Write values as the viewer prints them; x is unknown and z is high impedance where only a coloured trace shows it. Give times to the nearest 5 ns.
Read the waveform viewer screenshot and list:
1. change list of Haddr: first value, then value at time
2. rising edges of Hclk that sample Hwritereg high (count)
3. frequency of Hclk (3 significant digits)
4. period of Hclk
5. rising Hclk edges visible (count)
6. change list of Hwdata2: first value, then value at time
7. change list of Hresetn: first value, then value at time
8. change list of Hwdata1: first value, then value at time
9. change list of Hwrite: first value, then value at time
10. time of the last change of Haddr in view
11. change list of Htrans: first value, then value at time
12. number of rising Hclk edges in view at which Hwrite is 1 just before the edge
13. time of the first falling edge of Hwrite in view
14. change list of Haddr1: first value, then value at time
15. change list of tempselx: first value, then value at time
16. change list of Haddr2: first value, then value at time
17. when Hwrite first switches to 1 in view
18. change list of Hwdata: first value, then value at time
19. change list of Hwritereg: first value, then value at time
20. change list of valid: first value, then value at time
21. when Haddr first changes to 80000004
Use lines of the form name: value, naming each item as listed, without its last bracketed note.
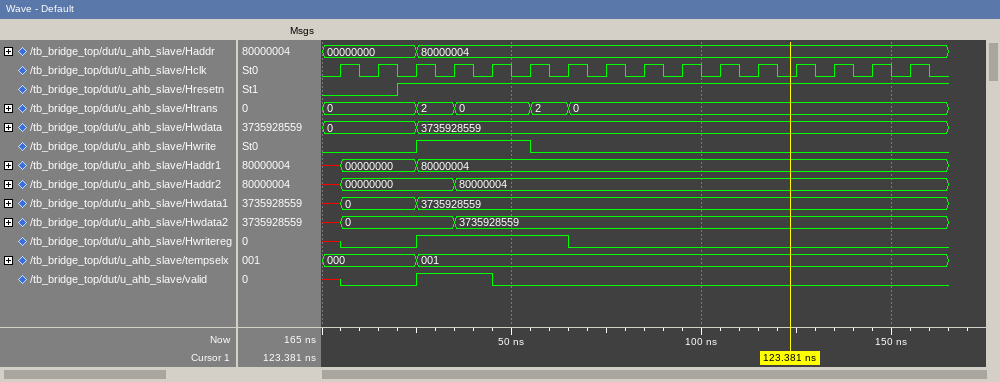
change list of Haddr: first value, then value at time: 00000000, 80000004 at 25 ns
rising edges of Hclk that sample Hwritereg high: 4
frequency of Hclk: 100 MHz
period of Hclk: 10 ns
rising Hclk edges visible: 16
change list of Hwdata2: first value, then value at time: x, 0 at 5 ns, 3735928559 at 35 ns
change list of Hresetn: first value, then value at time: 0, 1 at 20 ns
change list of Hwdata1: first value, then value at time: x, 0 at 5 ns, 3735928559 at 25 ns
change list of Hwrite: first value, then value at time: 0, 1 at 25 ns, 0 at 55 ns
time of the last change of Haddr in view: 25 ns
change list of Htrans: first value, then value at time: 0, 2 at 25 ns, 0 at 35 ns, 2 at 55 ns, 0 at 65 ns
number of rising Hclk edges in view at which Hwrite is 1 just before the edge: 3
time of the first falling edge of Hwrite in view: 55 ns
change list of Haddr1: first value, then value at time: x, 00000000 at 5 ns, 80000004 at 25 ns
change list of tempselx: first value, then value at time: 000, 001 at 25 ns
change list of Haddr2: first value, then value at time: x, 00000000 at 5 ns, 80000004 at 35 ns
when Hwrite first switches to 1 in view: 25 ns
change list of Hwdata: first value, then value at time: 0, 3735928559 at 25 ns
change list of Hwritereg: first value, then value at time: x, 0 at 5 ns, 1 at 25 ns, 0 at 65 ns
change list of valid: first value, then value at time: x, 0 at 5 ns, 1 at 25 ns, 0 at 45 ns
when Haddr first changes to 80000004: 25 ns
